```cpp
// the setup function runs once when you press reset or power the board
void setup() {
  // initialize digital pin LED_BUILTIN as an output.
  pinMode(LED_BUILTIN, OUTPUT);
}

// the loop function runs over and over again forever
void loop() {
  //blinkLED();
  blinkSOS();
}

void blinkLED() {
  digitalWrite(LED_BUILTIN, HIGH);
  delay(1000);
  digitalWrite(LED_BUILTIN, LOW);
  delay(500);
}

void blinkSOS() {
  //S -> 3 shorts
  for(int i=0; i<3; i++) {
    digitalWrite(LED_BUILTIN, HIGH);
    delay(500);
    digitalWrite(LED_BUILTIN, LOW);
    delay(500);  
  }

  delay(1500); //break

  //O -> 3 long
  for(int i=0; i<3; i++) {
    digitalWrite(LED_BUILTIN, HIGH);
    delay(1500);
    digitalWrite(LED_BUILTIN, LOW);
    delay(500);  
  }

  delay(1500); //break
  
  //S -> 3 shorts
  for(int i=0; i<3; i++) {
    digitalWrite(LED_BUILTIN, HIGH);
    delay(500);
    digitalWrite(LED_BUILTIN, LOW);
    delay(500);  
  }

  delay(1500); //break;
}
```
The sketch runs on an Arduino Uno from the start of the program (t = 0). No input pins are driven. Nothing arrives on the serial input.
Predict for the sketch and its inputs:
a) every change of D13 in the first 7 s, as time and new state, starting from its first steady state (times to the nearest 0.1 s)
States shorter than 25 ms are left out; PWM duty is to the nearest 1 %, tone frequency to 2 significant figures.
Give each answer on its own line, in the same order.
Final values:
0 s high; 0.5 s low; 1 s high; 1.5 s low; 2 s high; 2.5 s low; 4.5 s high; 6 s low; 6.5 s high
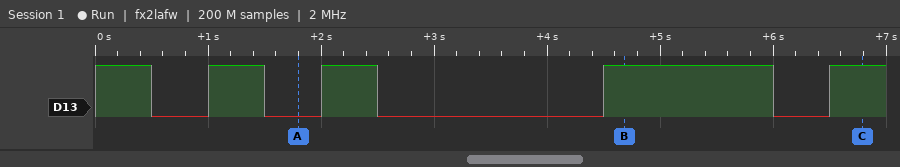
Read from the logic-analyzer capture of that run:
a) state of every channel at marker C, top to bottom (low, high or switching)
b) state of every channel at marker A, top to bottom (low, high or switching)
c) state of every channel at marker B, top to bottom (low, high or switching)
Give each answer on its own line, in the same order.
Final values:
D13 high
D13 low
D13 high
